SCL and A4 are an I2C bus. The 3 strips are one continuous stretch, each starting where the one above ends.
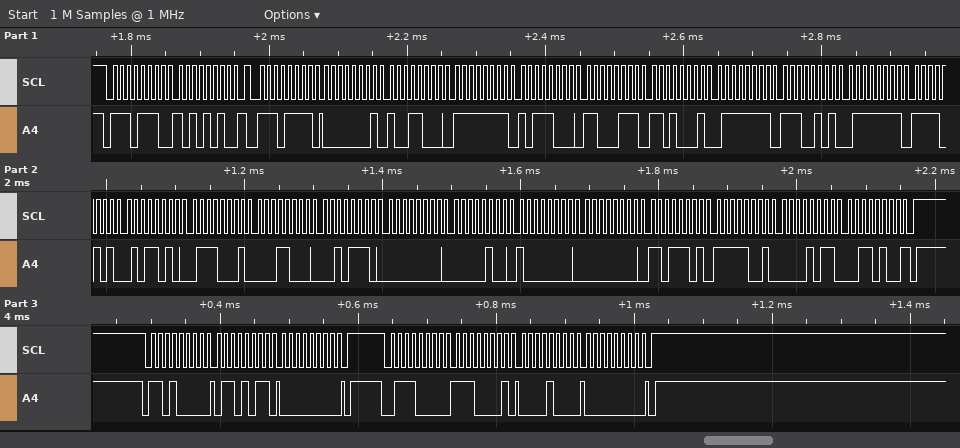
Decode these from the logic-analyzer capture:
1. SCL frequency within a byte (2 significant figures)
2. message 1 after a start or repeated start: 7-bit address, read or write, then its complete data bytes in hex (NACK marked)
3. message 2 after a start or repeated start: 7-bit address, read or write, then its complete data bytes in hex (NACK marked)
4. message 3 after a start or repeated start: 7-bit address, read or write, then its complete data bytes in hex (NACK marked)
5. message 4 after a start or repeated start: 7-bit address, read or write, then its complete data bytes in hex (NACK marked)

100 kHz
0x77 write: AA
0x77 read: 01 98 FF B8 C7 D1 7F E5 7F F5 5A 71 18 2E 00 04 80 00 DD F9 0B 34 NACK
0x68 write: 6B 00
0x38 write: E1 08 00
